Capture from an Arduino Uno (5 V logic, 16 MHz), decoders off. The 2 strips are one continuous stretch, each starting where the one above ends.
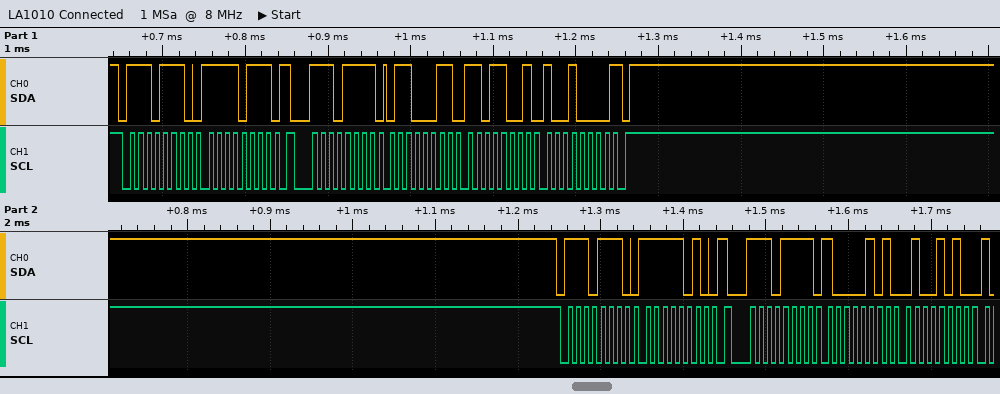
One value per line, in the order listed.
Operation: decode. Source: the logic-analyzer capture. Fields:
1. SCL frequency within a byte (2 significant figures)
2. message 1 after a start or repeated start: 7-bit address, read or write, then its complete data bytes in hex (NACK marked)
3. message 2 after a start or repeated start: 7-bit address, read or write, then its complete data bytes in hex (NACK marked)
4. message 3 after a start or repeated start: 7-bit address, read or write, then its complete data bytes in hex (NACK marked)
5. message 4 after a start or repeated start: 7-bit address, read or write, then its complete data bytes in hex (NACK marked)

100 kHz
0x77 write: F7
0x77 read: 63 D9 90 NACK
0x77 write: FA
0x77 read: 85 4A
